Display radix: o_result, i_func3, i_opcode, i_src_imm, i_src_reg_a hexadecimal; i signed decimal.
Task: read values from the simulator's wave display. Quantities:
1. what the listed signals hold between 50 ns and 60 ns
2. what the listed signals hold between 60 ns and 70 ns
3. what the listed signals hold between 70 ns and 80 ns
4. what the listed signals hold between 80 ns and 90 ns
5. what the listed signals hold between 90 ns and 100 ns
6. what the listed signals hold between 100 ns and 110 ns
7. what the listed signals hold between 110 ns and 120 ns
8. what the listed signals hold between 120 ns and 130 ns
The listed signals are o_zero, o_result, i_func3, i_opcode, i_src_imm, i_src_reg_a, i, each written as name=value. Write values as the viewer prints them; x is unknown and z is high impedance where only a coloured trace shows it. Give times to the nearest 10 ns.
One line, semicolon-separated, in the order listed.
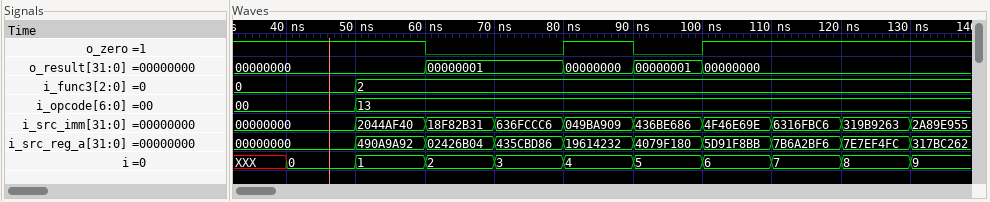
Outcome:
o_zero=1, o_result=00000000, i_func3=2, i_opcode=13, i_src_imm=2044AF40, i_src_reg_a=490A9A92, i=1; o_zero=0, o_result=00000001, i_func3=2, i_opcode=13, i_src_imm=18F82B31, i_src_reg_a=02426B04, i=2; o_zero=0, o_result=00000001, i_func3=2, i_opcode=13, i_src_imm=636FCCC6, i_src_reg_a=435CBD86, i=3; o_zero=1, o_result=00000000, i_func3=2, i_opcode=13, i_src_imm=049BA909, i_src_reg_a=19614232, i=4; o_zero=0, o_result=00000001, i_func3=2, i_opcode=13, i_src_imm=436BE686, i_src_reg_a=4079F180, i=5; o_zero=1, o_result=00000000, i_func3=2, i_opcode=13, i_src_imm=4F46E69E, i_src_reg_a=5D91F8BB, i=6; o_zero=1, o_result=00000000, i_func3=2, i_opcode=13, i_src_imm=6316FBC6, i_src_reg_a=7B6A2BF6, i=7; o_zero=1, o_result=00000000, i_func3=2, i_opcode=13, i_src_imm=319B9263, i_src_reg_a=7E7EF4FC, i=8
